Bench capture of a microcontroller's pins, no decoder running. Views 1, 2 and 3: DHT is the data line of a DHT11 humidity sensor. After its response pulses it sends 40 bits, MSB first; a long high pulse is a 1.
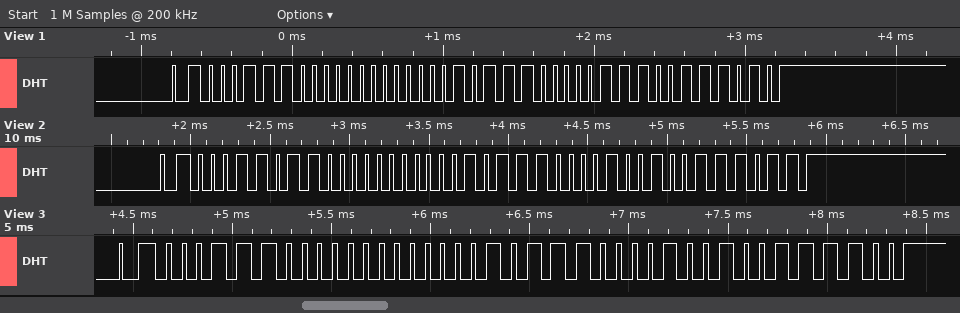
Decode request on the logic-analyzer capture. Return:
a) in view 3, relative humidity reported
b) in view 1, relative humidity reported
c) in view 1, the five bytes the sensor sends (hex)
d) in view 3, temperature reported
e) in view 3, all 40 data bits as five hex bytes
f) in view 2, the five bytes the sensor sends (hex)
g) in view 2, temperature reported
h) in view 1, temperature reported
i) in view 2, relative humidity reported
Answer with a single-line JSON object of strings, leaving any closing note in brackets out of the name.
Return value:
{"in view 3, relative humidity reported": "28 %", "in view 1, relative humidity reported": "28 %", "in view 1, the five bytes the sensor sends": "1C 00 17 07 3A", "in view 3, temperature reported": "23.9 °C", "in view 3, all 40 data bits as five hex bytes": "1C 00 17 09 3C", "in view 2, the five bytes the sensor sends": "1B 00 17 09 3B", "in view 2, temperature reported": "23.9 °C", "in view 1, temperature reported": "23.7 °C", "in view 2, relative humidity reported": "27 %"}
